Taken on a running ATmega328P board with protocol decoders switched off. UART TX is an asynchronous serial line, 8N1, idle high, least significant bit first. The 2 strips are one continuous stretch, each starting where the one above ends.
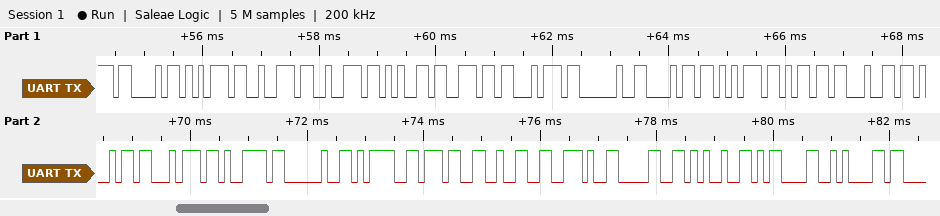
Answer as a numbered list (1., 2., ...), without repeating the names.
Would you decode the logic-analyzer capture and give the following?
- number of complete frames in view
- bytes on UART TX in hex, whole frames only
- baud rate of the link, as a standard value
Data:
1. 24
2. 43 75 72 72 65 6E 74 20 68 75 6D 64 69 74 79 20 3D 37 32 2E 30 25 0D 0A
3. 9600 baud
